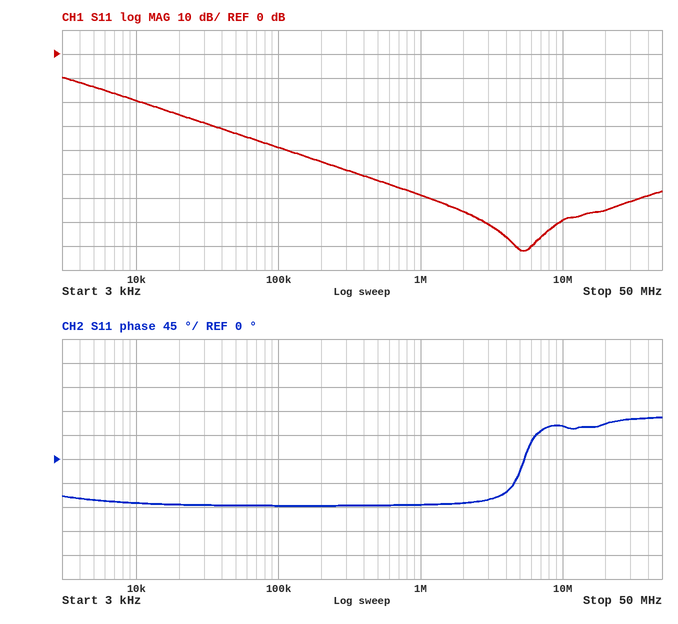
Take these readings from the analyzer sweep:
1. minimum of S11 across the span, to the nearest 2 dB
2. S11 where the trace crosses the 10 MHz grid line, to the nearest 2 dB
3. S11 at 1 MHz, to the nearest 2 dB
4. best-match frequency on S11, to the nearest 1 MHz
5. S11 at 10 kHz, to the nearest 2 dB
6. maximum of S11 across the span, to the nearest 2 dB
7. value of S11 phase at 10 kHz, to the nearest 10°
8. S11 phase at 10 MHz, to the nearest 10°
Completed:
-82 dB
-70 dB
-58 dB
5 MHz
-20 dB
-10 dB
-80°
60°
